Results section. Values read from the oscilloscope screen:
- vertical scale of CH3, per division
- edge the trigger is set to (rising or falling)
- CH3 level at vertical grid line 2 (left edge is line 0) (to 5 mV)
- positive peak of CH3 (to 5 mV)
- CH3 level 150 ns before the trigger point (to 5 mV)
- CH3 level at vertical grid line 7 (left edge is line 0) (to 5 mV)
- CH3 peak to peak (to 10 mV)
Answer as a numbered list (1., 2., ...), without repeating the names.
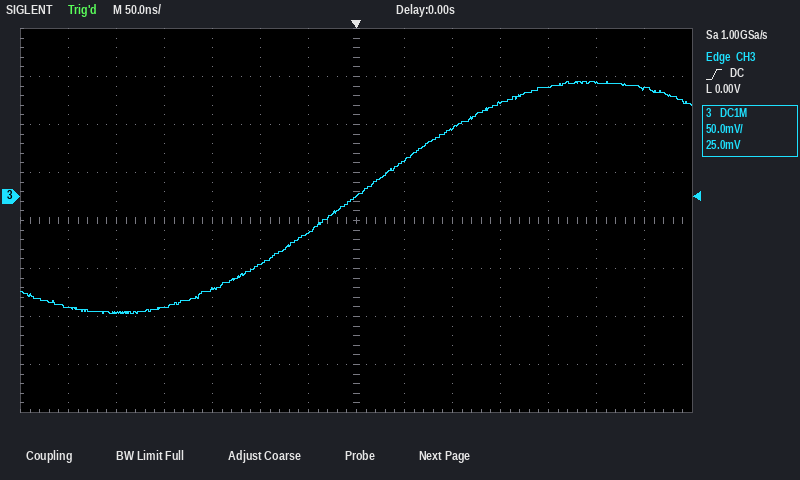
1. 50 mV
2. rising
3. -120 mV
4. 120 mV
5. -95 mV
6. 0 mV
7. 240 mV
